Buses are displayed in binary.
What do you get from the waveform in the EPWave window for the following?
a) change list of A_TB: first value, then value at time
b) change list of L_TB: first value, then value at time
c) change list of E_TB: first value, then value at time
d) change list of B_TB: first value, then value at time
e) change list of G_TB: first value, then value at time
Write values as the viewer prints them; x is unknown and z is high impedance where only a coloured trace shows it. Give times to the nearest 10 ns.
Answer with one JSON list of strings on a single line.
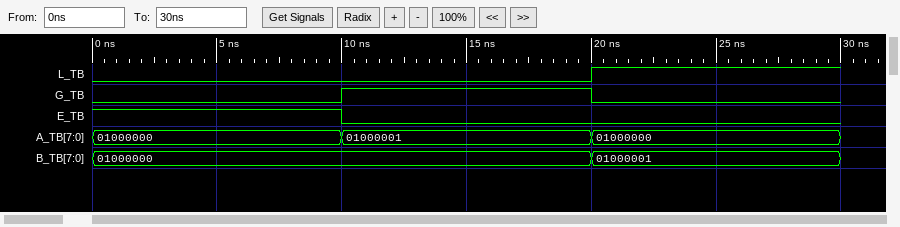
["01000000, 01000001 at 10 ns, 01000000 at 20 ns", "0, 1 at 20 ns", "1, 0 at 10 ns", "01000000, 01000001 at 20 ns", "0, 1 at 10 ns, 0 at 20 ns"]
